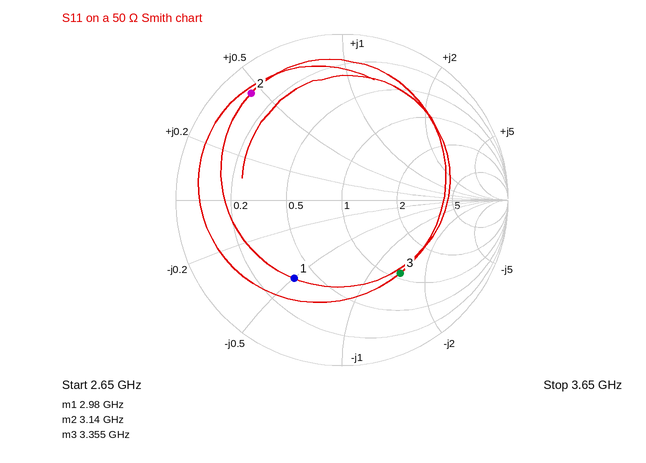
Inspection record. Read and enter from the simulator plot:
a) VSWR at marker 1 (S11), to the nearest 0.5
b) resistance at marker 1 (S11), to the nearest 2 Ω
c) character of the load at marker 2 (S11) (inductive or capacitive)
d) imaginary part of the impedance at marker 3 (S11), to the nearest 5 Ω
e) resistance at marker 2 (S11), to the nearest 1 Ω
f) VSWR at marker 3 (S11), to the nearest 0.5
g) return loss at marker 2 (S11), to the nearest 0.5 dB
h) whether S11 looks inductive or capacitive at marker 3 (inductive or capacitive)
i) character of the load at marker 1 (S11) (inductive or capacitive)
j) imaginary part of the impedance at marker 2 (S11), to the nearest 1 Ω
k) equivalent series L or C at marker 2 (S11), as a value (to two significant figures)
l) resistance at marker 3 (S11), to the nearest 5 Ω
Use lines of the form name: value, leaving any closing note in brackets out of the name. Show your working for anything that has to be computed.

VSWR at marker 1 (S11), to the nearest 0.5: 3.5
resistance at marker 1 (S11), to the nearest 2 Ω: 18 Ω
character of the load at marker 2 (S11): inductive
imaginary part of the impedance at marker 3 (S11), to the nearest 5 Ω: -70 Ω
resistance at marker 2 (S11), to the nearest 1 Ω: 5 Ω
VSWR at marker 3 (S11), to the nearest 0.5: 3.5
return loss at marker 2 (S11), to the nearest 0.5 dB: 1.5 dB
whether S11 looks inductive or capacitive at marker 3: capacitive
character of the load at marker 1 (S11): capacitive
imaginary part of the impedance at marker 2 (S11), to the nearest 1 Ω: +23 Ω
equivalent series L or C at marker 2 (S11), as a value: L = 23 Ω/(2π × 3.14 GHz) ≈ 1.2 nH
resistance at marker 3 (S11), to the nearest 5 Ω: 55 Ω
